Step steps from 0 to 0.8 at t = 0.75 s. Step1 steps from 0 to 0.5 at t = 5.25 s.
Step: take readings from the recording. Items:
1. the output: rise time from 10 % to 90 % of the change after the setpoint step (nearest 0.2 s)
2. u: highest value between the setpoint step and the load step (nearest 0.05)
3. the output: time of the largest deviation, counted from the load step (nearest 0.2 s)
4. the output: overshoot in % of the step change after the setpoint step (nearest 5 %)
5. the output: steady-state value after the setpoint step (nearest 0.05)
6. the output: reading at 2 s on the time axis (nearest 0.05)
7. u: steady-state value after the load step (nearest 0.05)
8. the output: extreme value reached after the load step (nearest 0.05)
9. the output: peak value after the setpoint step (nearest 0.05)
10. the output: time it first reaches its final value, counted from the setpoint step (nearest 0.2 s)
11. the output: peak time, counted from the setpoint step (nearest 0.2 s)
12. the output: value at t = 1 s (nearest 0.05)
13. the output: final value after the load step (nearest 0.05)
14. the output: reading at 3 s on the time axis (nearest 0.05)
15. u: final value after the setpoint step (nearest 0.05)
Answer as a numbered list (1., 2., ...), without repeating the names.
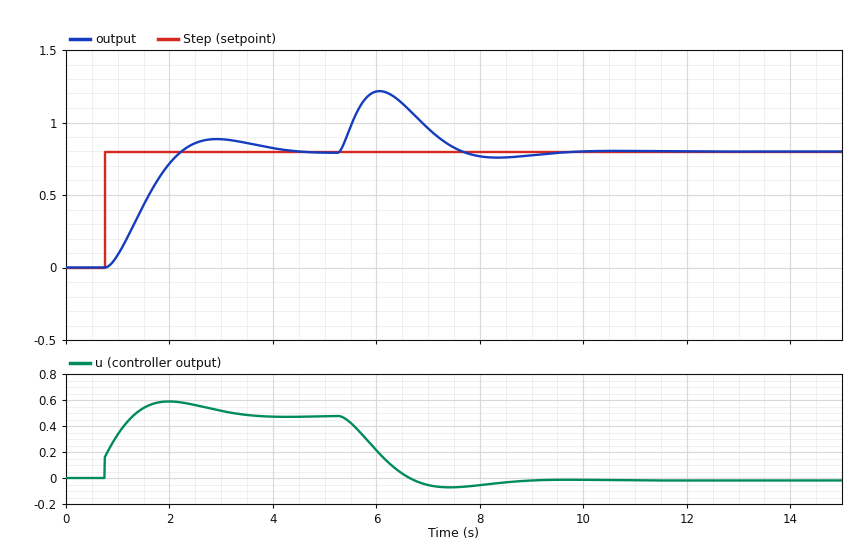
1. 1.0 s
2. 0.60
3. 0.8 s
4. 10 %
5. 0.80
6. 0.70
7. 0.00
8. 1.20
9. 0.90
10. 1.4 s
11. 2.2 s
12. 0.10
13. 0.80
14. 0.90
15. 0.50
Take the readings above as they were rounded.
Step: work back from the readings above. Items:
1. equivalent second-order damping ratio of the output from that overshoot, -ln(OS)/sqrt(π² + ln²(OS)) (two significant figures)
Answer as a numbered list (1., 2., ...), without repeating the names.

1. 0.59
